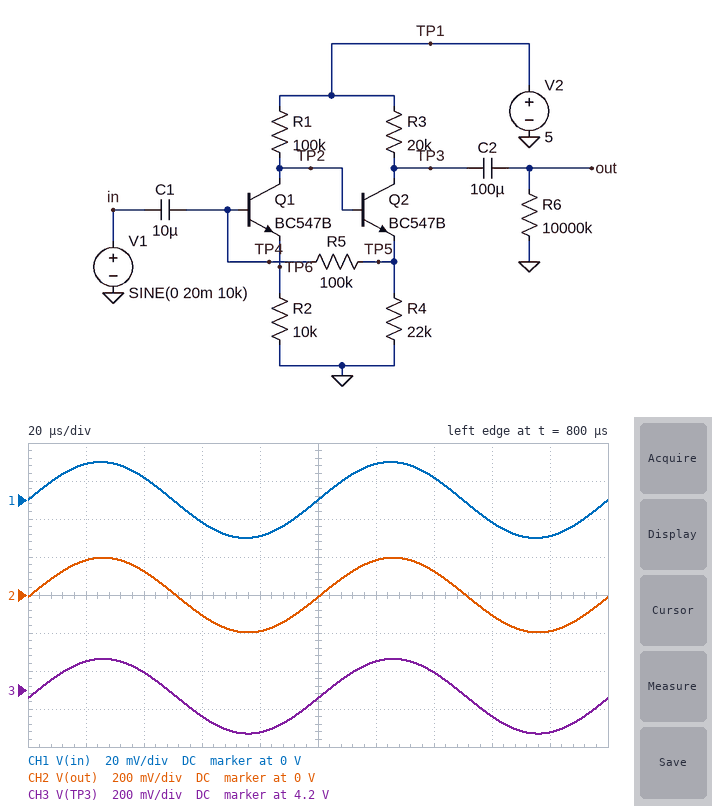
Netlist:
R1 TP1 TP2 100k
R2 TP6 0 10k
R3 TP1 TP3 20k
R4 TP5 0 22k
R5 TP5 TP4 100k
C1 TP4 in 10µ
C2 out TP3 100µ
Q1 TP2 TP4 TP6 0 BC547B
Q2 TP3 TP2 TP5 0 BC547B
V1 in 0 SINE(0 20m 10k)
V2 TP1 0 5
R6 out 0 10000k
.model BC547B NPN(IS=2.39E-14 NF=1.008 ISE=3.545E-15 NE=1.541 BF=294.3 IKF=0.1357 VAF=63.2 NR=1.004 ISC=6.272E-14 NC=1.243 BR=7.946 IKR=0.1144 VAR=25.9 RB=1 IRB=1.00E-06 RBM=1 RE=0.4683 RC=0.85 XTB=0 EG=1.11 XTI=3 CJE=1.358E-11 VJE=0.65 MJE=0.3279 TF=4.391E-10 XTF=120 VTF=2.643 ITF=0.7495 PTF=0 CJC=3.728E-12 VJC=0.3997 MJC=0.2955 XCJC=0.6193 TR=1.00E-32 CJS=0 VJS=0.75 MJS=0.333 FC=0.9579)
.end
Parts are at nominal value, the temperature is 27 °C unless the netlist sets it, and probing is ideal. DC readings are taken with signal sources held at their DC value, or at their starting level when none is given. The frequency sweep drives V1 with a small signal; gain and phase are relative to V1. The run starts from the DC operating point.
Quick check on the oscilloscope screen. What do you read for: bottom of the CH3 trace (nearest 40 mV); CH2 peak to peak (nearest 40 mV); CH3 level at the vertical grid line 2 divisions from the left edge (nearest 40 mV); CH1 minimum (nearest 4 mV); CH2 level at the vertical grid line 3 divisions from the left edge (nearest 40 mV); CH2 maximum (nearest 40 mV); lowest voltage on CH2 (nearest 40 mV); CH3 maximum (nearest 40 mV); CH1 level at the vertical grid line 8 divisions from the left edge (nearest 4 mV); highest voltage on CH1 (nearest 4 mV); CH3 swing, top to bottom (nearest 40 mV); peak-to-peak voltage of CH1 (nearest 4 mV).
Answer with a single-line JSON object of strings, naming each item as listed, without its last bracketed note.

{"bottom of the CH3 trace": "3.96 V", "CH2 peak to peak": "400 mV", "CH3 level at the vertical grid line 2 divisions from the left edge": "4.28 V", "CH1 minimum": "-20 mV", "CH2 level at the vertical grid line 3 divisions from the left edge": "-120 mV", "CH2 maximum": "200 mV", "lowest voltage on CH2": "-200 mV", "CH3 maximum": "4.36 V", "CH1 level at the vertical grid line 8 divisions from the left edge": "-12 mV", "highest voltage on CH1": "20 mV", "CH3 swing, top to bottom": "400 mV", "peak-to-peak voltage of CH1": "40 mV"}
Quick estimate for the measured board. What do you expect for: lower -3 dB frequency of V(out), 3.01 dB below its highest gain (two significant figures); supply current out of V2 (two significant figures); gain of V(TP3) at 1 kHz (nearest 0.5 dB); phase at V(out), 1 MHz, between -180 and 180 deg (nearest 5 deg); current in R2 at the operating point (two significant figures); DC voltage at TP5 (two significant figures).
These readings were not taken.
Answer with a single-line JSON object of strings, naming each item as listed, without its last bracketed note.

{"lower -3 dB frequency of V(out), 3.01 dB below its highest gain": "1.6 Hz", "supply current out of V2": "77 µA", "gain of V(TP3) at 1 kHz": "20.0 dB", "phase at V(out), 1 MHz, between -180 and 180 deg": "-115 deg", "current in R2 at the operating point": "35 µA", "DC voltage at TP5": "920 mV"}
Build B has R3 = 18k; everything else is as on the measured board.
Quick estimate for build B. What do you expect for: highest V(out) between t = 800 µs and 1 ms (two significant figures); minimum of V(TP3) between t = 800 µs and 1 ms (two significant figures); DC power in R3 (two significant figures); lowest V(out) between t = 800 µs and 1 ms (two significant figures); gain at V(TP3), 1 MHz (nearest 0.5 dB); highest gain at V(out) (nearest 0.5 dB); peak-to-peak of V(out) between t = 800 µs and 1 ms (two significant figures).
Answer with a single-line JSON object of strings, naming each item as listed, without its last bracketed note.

{"highest V(out) between t = 800 µs and 1 ms": "180 mV", "minimum of V(TP3) between t = 800 µs and 1 ms": "4.1 V", "DC power in R3": "31 µW", "lowest V(out) between t = 800 µs and 1 ms": "-180 mV", "gain at V(TP3), 1 MHz": "5.5 dB", "highest gain at V(out)": "19.0 dB", "peak-to-peak of V(out) between t = 800 µs and 1 ms": "350 mV"}
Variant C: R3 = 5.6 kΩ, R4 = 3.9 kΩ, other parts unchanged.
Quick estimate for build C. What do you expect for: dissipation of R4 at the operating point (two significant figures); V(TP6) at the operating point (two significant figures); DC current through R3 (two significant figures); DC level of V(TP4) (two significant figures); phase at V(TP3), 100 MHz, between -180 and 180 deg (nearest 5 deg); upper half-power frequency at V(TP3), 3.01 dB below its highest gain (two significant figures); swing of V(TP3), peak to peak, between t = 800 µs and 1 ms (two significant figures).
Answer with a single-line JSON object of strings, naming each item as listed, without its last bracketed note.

{"dissipation of R4 at the operating point": "210 µW", "V(TP6) at the operating point": "340 mV", "DC current through R3": "230 µA", "DC level of V(TP4)": "890 mV", "phase at V(TP3), 100 MHz, between -180 and 180 deg": "25 deg", "upper half-power frequency at V(TP3), 3.01 dB below its highest gain": "190 kHz", "swing of V(TP3), peak to peak, between t = 800 µs and 1 ms": "490 mV"}
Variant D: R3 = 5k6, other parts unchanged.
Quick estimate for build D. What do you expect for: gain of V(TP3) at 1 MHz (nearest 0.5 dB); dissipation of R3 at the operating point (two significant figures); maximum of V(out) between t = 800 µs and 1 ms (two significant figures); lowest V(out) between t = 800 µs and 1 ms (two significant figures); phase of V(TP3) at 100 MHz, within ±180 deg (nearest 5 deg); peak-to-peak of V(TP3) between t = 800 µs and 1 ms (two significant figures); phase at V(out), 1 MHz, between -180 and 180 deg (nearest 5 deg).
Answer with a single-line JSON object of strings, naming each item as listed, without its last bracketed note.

{"gain of V(TP3) at 1 MHz": "-3.0 dB", "dissipation of R3 at the operating point": "9.7 µW", "maximum of V(out) between t = 800 µs and 1 ms": "55 mV", "lowest V(out) between t = 800 µs and 1 ms": "-55 mV", "phase of V(TP3) at 100 MHz, within ±180 deg": "15 deg", "peak-to-peak of V(TP3) between t = 800 µs and 1 ms": "110 mV", "phase at V(out), 1 MHz, between -180 and 180 deg": "-110 deg"}
